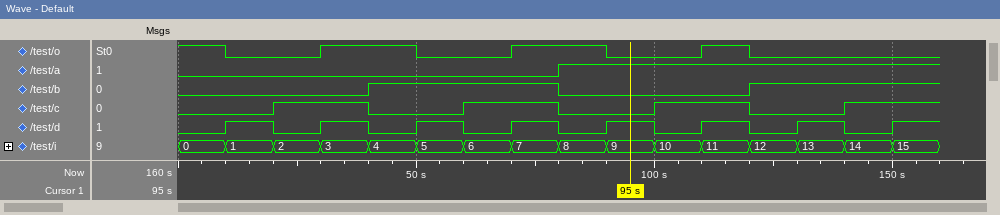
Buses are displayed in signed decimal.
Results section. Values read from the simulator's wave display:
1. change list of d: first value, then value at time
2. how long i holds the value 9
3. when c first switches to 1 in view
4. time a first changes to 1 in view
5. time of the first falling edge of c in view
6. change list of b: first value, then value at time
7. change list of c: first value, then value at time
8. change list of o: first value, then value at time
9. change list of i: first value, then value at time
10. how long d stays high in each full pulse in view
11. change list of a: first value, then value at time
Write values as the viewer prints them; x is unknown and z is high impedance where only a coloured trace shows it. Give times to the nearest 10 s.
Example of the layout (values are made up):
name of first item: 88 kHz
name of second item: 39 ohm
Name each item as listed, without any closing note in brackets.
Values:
change list of d: first value, then value at time: 0, 1 at 10 s, 0 at 20 s, 1 at 30 s, 0 at 40 s, 1 at 50 s, 0 at 60 s, 1 at 70 s, 0 at 80 s, 1 at 90 s, 0 at 100 s, 1 at 110 s, 0 at 120 s, 1 at 130 s, 0 at 140 s, 1 at 150 s
how long i holds the value 9: 10 s
when c first switches to 1 in view: 20 s
time a first changes to 1 in view: 80 s
time of the first falling edge of c in view: 40 s
change list of b: first value, then value at time: 0, 1 at 40 s, 0 at 80 s, 1 at 120 s
change list of c: first value, then value at time: 0, 1 at 20 s, 0 at 40 s, 1 at 60 s, 0 at 80 s, 1 at 100 s, 0 at 120 s, 1 at 140 s
change list of o: first value, then value at time: 1, 0 at 10 s, 1 at 30 s, 0 at 50 s, 1 at 70 s, 0 at 90 s, 1 at 110 s, 0 at 120 s
change list of i: first value, then value at time: 0, 1 at 10 s, 2 at 20 s, 3 at 30 s, 4 at 40 s, 5 at 50 s, 6 at 60 s, 7 at 70 s, 8 at 80 s, 9 at 90 s, 10 at 100 s, 11 at 110 s, 12 at 120 s, 13 at 130 s, 14 at 140 s, 15 at 150 s
how long d stays high in each full pulse in view: 10 s, 10 s, 10 s, 10 s, 10 s, 10 s, 10 s
change list of a: first value, then value at time: 0, 1 at 80 s
